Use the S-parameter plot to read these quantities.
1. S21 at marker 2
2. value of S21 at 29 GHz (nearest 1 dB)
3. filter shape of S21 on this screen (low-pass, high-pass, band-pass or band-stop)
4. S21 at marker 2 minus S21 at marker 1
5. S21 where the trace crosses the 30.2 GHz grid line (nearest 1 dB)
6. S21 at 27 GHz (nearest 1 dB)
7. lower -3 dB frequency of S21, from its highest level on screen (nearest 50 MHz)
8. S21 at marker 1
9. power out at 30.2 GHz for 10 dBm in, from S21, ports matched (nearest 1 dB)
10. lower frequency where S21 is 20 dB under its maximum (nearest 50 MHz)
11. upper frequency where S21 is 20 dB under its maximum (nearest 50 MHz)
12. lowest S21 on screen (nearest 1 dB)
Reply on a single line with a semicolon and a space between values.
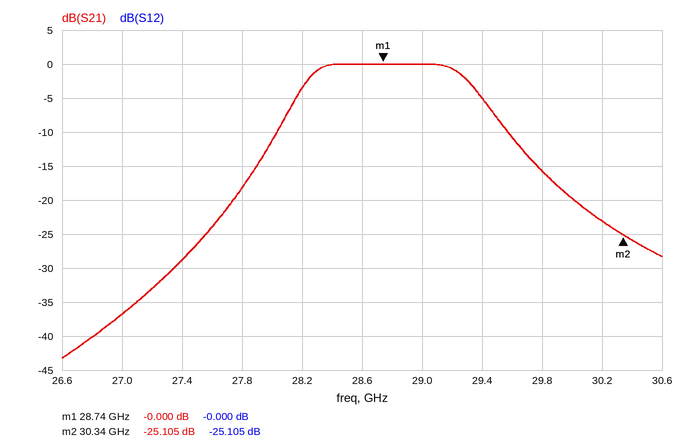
-25.105 dB; 0 dB; band-pass; -25.105 dB; -23 dB; -37 dB; 28.20 GHz; -0.000 dB; -13 dBm; 27.75 GHz; 30.00 GHz; -43 dB
